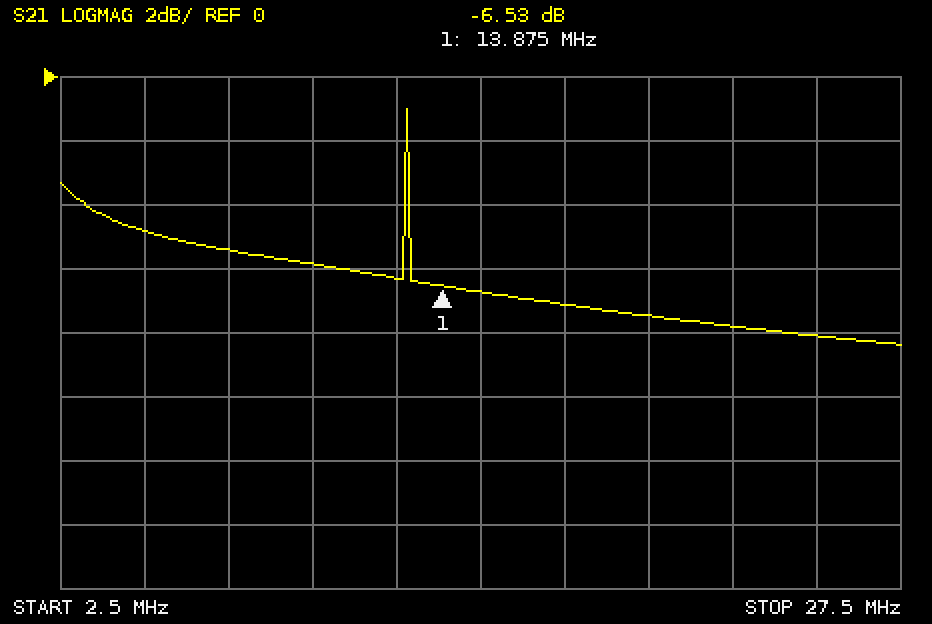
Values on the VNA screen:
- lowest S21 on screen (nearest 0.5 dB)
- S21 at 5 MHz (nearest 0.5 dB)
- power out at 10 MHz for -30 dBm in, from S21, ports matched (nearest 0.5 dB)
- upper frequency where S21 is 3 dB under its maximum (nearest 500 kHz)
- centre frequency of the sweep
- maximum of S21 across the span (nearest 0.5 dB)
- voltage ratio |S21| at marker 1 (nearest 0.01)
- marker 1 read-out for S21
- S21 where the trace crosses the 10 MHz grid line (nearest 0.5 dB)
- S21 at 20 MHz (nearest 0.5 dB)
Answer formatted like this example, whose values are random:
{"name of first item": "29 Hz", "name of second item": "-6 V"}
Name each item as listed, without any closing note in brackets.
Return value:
{"lowest S21 on screen": "-8.5 dB", "S21 at 5 MHz": "-5.0 dB", "power out at 10 MHz for -30 dBm in, from S21, ports matched": "-36.0 dBm", "upper frequency where S21 is 3 dB under its maximum": "13.0 MHz", "centre frequency of the sweep": "15 MHz", "maximum of S21 across the span": "-1.0 dB", "voltage ratio |S21| at marker 1": "0.47", "marker 1 read-out for S21": "-6.53 dB", "S21 where the trace crosses the 10 MHz grid line": "-6.0 dB", "S21 at 20 MHz": "-7.5 dB"}
